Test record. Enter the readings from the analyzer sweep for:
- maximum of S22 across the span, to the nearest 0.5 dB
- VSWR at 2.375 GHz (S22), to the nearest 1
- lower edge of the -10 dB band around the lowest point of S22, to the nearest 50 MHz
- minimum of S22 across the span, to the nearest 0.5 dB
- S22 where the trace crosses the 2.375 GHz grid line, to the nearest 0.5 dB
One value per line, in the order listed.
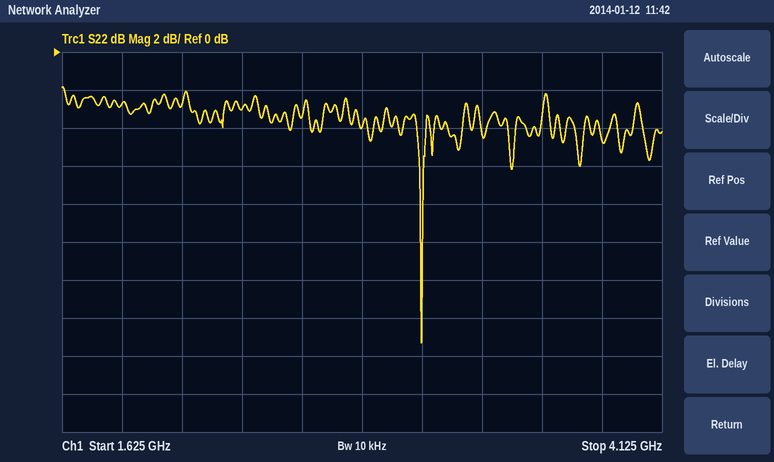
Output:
-2.0 dB
6
3.10 GHz
-15.5 dB
-3.0 dB
